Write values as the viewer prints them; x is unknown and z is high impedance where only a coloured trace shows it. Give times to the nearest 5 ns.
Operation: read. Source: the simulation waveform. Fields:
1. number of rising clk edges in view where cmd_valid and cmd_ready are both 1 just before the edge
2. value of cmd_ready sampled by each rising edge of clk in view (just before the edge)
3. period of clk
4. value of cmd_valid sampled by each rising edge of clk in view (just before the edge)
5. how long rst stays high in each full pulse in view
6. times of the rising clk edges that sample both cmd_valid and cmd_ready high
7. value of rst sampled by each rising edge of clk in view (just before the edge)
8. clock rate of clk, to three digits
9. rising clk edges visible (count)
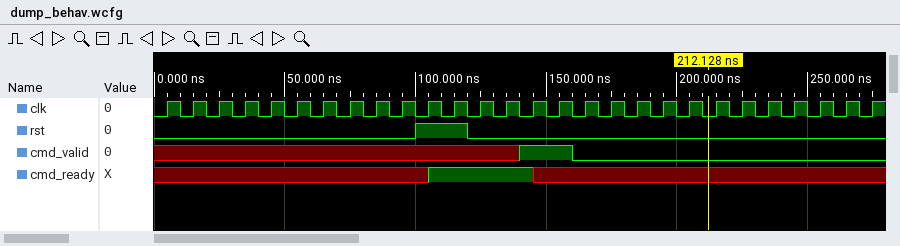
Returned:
1
x x x x x x x x x x x 1 1 1 1 x x x x x x x x x x x x x
10 ns
x x x x x x x x x x x x x x 1 1 0 0 0 0 0 0 0 0 0 0 0 0
20 ns
145 ns
0 0 0 0 0 0 0 0 0 0 1 1 0 0 0 0 0 0 0 0 0 0 0 0 0 0 0 0
100 MHz
28
